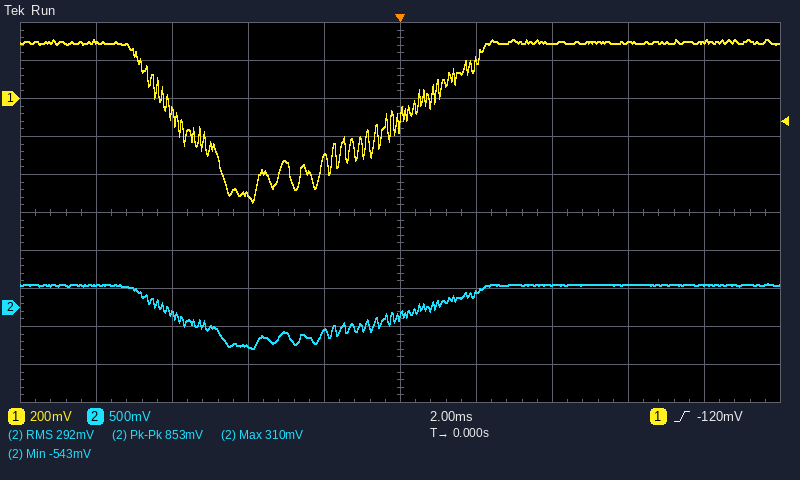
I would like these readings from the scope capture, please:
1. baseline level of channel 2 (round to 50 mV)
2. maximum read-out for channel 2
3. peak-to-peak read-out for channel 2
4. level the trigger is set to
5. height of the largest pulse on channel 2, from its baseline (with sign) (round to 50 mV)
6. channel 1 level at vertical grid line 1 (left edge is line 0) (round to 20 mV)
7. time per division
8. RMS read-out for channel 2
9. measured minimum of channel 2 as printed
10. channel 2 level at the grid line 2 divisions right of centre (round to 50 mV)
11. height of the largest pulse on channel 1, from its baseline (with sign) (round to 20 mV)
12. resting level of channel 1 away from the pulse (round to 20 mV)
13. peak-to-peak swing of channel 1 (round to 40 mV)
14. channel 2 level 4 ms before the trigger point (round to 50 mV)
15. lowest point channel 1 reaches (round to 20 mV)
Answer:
300 mV
310 mV
853 mV
-120 mV
-850 mV
300 mV
2 ms
292 mV
-543 mV
300 mV
-840 mV
300 mV
840 mV
-500 mV
-540 mV
